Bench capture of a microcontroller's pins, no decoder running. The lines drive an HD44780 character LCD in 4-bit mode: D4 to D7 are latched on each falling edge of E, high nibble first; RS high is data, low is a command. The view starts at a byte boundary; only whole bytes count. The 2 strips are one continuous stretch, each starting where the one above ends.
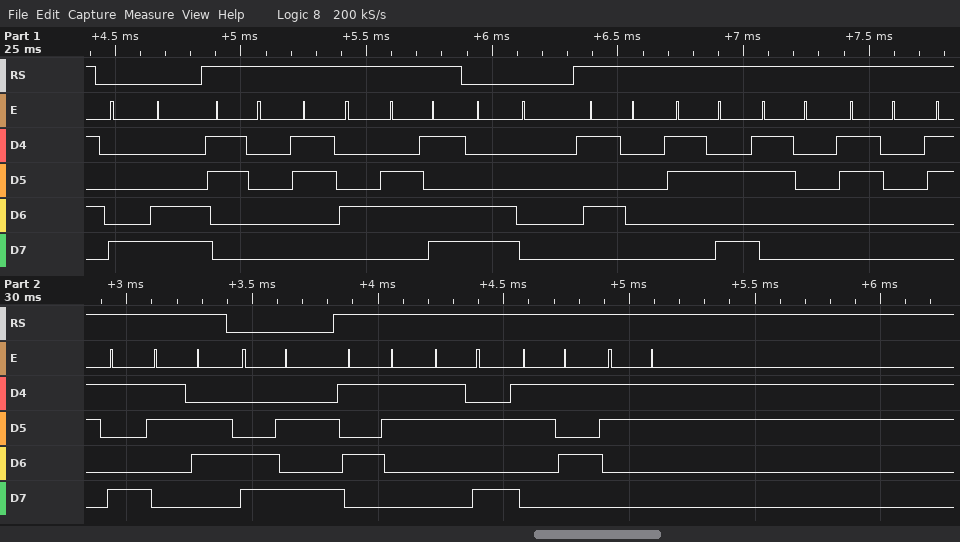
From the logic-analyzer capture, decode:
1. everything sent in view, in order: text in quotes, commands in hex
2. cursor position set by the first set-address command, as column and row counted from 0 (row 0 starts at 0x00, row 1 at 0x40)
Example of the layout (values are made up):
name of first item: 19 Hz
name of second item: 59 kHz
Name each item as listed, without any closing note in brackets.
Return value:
everything sent in view, in order: text in quotes, commands in hex: 0x8C "04m" 0xC0 "P:0096" 0xCA "S:53"
cursor position set by the first set-address command, as column and row counted from 0: column 12, row 0
